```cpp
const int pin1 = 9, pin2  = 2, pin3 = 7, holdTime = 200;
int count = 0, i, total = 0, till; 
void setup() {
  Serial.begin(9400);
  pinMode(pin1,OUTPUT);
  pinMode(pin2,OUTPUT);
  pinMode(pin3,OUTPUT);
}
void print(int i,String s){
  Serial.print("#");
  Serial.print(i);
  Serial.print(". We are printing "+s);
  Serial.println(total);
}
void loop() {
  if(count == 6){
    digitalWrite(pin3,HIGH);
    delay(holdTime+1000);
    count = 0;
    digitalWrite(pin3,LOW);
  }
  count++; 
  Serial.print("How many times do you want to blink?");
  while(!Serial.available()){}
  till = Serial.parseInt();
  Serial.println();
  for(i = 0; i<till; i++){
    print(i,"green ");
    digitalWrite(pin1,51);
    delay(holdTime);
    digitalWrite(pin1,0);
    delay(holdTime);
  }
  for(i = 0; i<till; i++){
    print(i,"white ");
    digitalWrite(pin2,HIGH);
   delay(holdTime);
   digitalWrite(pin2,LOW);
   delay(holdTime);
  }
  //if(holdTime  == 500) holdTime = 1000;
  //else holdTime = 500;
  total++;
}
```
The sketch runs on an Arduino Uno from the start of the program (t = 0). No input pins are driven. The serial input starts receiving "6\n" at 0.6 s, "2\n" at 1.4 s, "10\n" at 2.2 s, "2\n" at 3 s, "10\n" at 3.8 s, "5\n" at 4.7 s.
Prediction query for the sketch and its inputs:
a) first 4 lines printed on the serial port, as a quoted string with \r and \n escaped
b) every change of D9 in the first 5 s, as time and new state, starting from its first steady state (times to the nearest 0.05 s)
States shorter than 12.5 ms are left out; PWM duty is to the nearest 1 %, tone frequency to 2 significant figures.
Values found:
"How many times do you want to blink?\r\n#0. We are printing green 0\r\n#1. We are printing green 0\r\n#2. We are printing green 0\r\n"
0 s low; 0.6 s high; 0.8 s low; 1 s high; 1.2 s low; 1.4 s high; 1.6 s low; 1.8 s high; 2 s low; 2.2 s high; 2.4 s low; 2.6 s high; 2.8 s low
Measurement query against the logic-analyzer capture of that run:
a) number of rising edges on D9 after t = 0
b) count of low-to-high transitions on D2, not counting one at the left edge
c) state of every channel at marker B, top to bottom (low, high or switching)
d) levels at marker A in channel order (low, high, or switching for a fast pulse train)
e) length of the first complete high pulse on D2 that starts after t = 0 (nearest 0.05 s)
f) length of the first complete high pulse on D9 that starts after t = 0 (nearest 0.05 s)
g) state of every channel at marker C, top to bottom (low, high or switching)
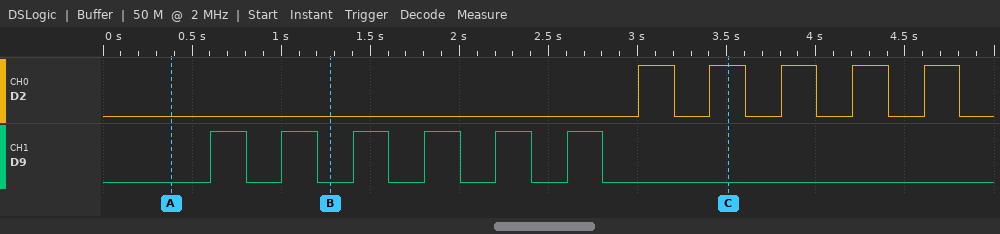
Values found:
6
5
D2 low, D9 low
D2 low, D9 low
0.20 s
0.20 s
D2 high, D9 low
